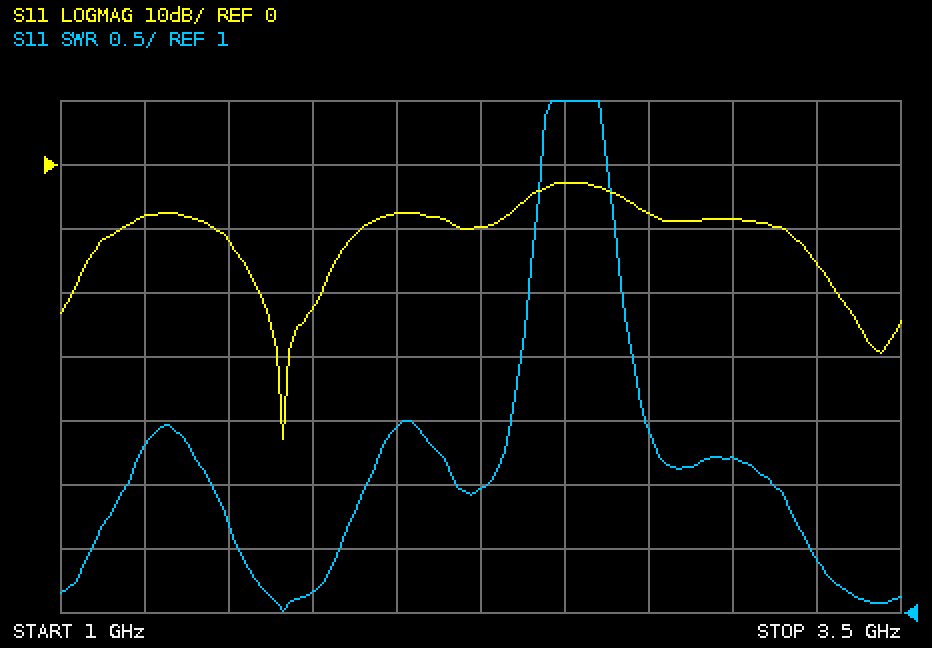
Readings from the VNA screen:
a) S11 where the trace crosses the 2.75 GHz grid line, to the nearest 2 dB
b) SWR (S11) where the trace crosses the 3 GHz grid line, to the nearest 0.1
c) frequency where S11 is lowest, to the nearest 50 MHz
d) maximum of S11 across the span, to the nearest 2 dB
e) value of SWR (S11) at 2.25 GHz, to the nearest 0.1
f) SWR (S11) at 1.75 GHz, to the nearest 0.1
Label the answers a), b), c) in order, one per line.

a) -8 dB
b) 2.2
c) 1.65 GHz
d) -2 dB
e) 2.0
f) 1.2
